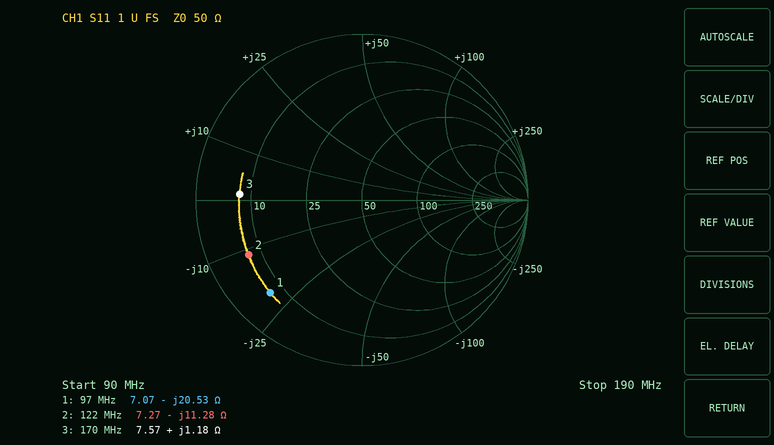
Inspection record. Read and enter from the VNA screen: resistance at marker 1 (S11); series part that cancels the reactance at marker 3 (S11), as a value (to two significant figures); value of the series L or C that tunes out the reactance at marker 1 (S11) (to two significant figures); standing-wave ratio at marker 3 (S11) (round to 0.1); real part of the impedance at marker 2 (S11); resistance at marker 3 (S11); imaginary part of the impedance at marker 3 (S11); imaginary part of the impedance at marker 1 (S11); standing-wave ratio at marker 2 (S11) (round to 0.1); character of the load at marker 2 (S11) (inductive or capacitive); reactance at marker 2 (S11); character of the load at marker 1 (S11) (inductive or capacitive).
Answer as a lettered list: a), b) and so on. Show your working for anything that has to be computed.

a) 7.07 Ω
b) C = 1/(2π × 170 MHz × 1.18 Ω) ≈ 793 pF, so 790 pF to two significant figures
c) L = 20.53 Ω/(2π × 97 MHz) ≈ 34 nH
d) 6.6
e) 7.27 Ω
f) 7.57 Ω
g) +1.18 Ω
h) -20.53 Ω
i) 7.2
j) capacitive
k) -11.28 Ω
l) capacitive
